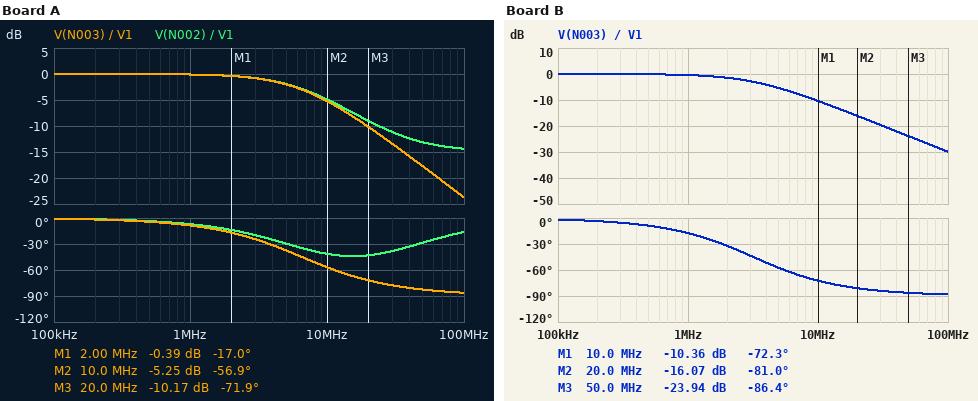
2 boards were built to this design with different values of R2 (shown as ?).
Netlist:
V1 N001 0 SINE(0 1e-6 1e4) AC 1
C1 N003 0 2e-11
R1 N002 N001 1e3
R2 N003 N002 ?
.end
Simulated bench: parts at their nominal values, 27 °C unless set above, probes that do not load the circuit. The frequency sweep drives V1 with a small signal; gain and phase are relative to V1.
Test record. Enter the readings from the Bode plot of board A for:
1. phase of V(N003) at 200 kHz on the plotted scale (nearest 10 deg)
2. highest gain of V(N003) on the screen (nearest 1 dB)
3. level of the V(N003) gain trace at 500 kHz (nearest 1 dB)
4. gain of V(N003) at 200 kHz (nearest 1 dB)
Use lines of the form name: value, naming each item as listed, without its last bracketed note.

phase of V(N003) at 200 kHz on the plotted scale: 0 deg
highest gain of V(N003) on the screen: 0 dB
level of the V(N003) gain trace at 500 kHz: 0 dB
gain of V(N003) at 200 kHz: 0 dB
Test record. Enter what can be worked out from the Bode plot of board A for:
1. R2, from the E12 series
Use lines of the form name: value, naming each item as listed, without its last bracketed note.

R2, from the E12 series: 220 Ω
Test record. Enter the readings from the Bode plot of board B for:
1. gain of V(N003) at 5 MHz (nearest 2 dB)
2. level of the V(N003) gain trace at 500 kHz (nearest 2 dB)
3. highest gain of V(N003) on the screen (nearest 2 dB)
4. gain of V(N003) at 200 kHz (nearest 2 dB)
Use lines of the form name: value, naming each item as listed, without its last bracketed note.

gain of V(N003) at 5 MHz: -6 dB
level of the V(N003) gain trace at 500 kHz: 0 dB
highest gain of V(N003) on the screen: 0 dB
gain of V(N003) at 200 kHz: 0 dB
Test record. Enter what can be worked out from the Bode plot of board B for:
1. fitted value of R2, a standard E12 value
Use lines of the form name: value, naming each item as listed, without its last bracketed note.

fitted value of R2, a standard E12 value: 1.5 kΩ
